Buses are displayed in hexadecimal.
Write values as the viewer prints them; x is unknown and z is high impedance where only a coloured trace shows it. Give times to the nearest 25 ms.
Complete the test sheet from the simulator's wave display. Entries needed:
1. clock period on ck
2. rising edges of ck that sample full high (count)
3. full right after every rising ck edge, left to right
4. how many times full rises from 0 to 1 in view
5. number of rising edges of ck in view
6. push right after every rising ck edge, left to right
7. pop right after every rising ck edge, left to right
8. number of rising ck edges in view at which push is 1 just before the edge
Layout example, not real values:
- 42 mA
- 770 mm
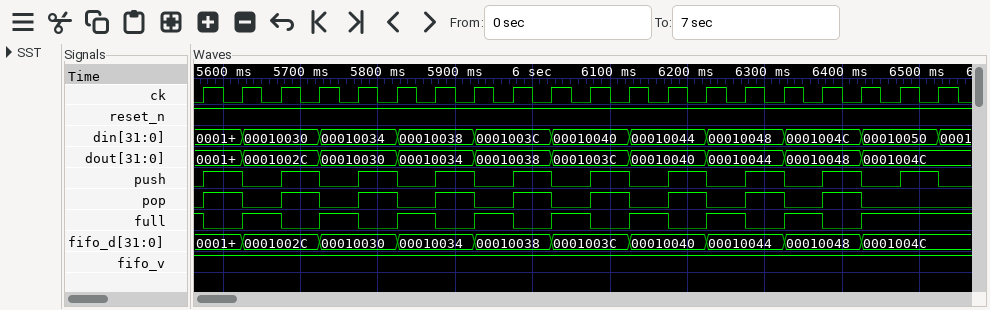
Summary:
- 50 ms
- 11
- 0 1 0 1 0 1 0 1 0 1 0 1 0 1 0 1 0 1 1 1
- 9
- 20
- 1 0 1 0 1 0 1 0 1 0 1 0 1 0 1 0 1 0 1 0
- 1 0 1 0 1 0 1 0 1 0 1 0 1 0 1 0 1 0 0 0
- 10
